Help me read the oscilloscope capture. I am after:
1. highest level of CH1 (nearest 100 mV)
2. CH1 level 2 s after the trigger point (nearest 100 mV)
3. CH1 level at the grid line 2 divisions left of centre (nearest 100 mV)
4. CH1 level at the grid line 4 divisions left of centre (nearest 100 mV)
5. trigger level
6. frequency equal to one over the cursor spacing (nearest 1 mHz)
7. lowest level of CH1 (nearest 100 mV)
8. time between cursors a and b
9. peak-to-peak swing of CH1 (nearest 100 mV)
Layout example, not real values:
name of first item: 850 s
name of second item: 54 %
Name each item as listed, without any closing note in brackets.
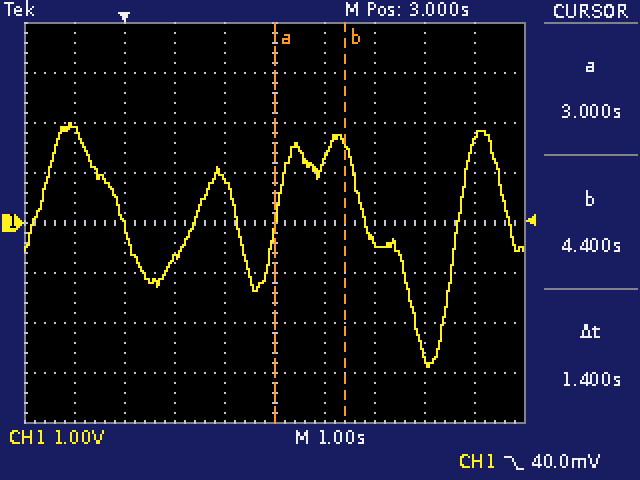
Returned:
highest level of CH1: 2.0 V
CH1 level 2 s after the trigger point: 900 mV
CH1 level at the grid line 2 divisions left of centre: -700 mV
CH1 level at the grid line 4 divisions left of centre: 1.9 V
trigger level: 40.0 mV
frequency equal to one over the cursor spacing: 714 mHz
lowest level of CH1: -2.9 V
time between cursors a and b: 1.4 s
peak-to-peak swing of CH1: 4.9 V
